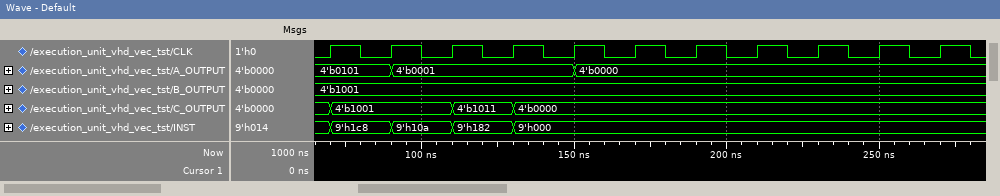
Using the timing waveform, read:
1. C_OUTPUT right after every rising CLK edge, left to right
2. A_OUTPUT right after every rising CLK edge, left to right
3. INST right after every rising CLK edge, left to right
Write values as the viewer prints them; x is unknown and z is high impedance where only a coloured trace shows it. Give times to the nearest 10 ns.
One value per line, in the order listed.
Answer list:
4'b1001, 4'b1001, 4'b1011, 4'b0000, 4'b0000, 4'b0000, 4'b0000, 4'b0000, 4'b0000, 4'b0000, 4'b0000
4'b0101, 4'b0001, 4'b0001, 4'b0001, 4'b0000, 4'b0000, 4'b0000, 4'b0000, 4'b0000, 4'b0000, 4'b0000
9'h1c8, 9'h10a, 9'h182, 9'h000, 9'h000, 9'h000, 9'h000, 9'h000, 9'h000, 9'h000, 9'h000
